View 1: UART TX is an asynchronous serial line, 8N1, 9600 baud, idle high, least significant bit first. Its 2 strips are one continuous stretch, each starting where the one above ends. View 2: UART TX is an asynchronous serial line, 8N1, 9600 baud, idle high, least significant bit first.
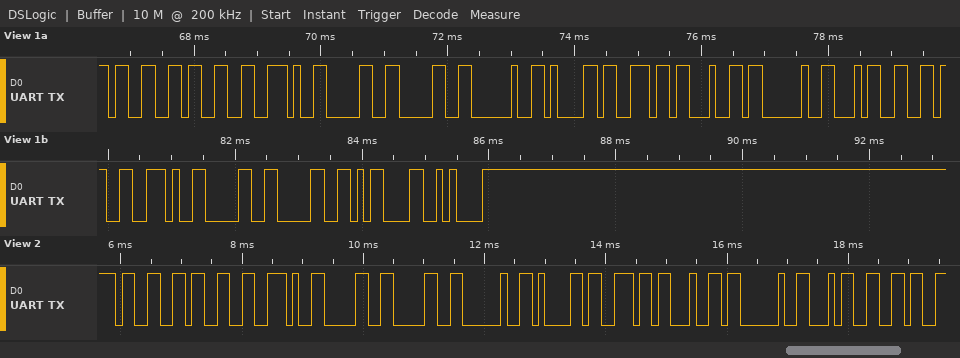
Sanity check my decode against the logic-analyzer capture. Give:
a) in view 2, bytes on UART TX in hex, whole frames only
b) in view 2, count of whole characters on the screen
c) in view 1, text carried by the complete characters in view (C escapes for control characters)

0x33 0x33 0x2E 0x30 0x30 0x20 0x61 0x6E 0x64 0x20 0x34 0x36
12
"33.00 and 46.00\r\n"
